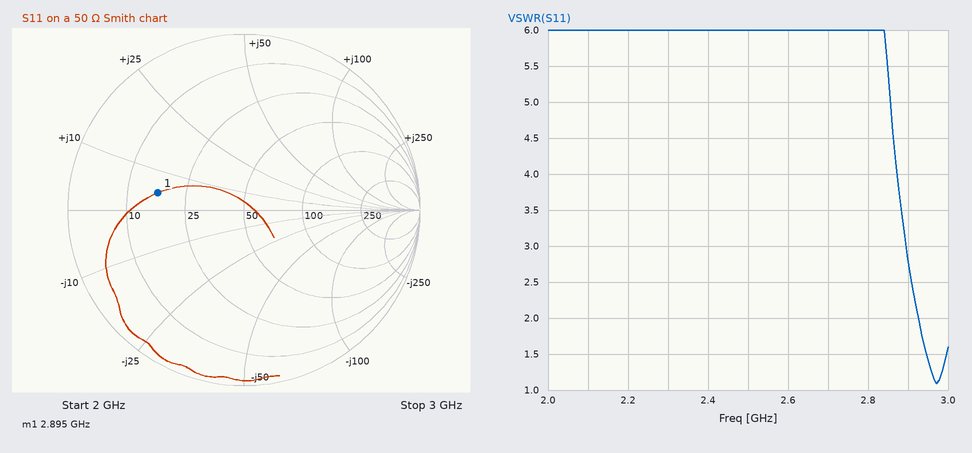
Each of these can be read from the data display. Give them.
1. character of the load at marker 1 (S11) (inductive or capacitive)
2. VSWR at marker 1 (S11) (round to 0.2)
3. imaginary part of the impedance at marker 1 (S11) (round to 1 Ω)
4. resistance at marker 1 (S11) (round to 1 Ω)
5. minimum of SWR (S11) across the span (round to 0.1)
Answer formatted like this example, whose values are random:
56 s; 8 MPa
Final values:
inductive; 3.0; +4 Ω; 17 Ω; 1.1
